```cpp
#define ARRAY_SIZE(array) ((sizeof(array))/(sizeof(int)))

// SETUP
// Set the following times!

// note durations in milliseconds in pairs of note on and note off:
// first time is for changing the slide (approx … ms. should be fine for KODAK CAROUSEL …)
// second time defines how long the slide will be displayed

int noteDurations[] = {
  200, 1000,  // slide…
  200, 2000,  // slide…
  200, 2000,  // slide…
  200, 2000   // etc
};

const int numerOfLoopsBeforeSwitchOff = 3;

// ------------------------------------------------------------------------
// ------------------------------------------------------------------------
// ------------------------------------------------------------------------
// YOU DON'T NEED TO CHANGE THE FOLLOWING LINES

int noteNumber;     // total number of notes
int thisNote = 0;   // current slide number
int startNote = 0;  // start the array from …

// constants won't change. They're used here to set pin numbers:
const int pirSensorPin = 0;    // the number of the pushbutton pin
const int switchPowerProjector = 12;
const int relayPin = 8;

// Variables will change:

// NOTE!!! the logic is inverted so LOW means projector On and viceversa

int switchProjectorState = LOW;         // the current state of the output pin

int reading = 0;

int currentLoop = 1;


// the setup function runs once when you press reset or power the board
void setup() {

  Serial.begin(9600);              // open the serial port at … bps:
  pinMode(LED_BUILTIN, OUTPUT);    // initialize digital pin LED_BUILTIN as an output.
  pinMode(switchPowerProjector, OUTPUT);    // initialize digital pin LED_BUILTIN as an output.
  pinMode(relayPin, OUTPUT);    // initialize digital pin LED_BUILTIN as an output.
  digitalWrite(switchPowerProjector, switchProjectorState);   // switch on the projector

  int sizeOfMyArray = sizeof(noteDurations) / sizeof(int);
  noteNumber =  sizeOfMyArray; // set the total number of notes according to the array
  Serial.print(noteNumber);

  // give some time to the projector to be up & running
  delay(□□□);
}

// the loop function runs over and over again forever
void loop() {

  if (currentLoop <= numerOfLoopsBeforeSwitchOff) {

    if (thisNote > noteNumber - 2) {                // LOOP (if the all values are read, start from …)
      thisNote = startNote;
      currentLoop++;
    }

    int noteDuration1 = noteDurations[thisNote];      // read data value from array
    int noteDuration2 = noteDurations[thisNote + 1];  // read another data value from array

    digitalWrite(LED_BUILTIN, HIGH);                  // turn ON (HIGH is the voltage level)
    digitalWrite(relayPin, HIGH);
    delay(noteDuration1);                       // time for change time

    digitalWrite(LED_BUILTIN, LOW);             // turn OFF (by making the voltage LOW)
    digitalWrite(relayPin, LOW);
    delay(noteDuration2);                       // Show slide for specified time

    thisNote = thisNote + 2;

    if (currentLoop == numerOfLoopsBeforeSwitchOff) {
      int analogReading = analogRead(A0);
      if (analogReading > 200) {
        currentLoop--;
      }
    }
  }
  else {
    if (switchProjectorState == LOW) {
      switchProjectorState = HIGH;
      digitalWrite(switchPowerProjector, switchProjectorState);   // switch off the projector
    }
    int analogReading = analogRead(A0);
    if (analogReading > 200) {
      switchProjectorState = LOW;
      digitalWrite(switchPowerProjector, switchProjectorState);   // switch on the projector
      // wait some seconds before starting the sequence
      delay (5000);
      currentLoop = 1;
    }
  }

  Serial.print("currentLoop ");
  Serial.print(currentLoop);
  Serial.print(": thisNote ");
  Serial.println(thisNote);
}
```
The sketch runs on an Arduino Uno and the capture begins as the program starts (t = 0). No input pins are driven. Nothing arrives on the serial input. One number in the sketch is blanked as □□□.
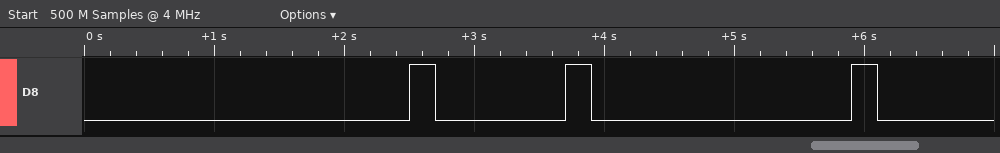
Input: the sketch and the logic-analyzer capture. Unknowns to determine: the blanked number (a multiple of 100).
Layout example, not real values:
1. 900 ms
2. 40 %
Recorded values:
1. 2500
